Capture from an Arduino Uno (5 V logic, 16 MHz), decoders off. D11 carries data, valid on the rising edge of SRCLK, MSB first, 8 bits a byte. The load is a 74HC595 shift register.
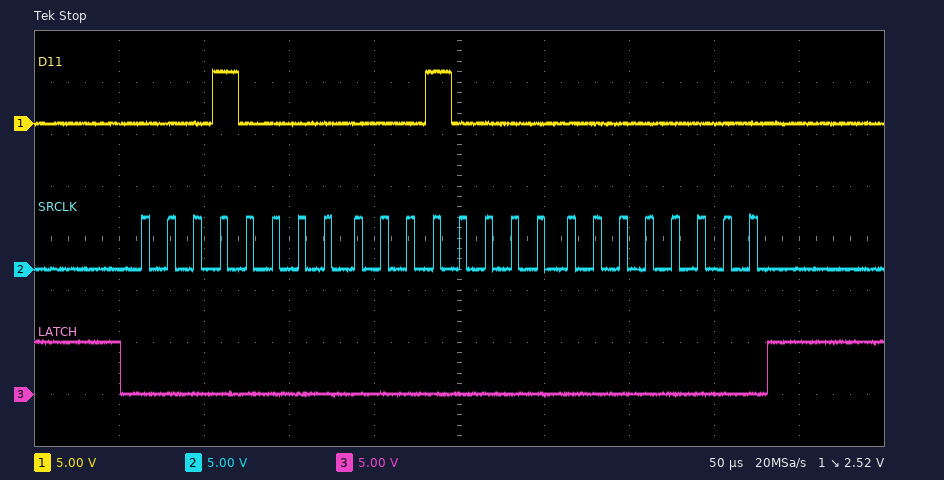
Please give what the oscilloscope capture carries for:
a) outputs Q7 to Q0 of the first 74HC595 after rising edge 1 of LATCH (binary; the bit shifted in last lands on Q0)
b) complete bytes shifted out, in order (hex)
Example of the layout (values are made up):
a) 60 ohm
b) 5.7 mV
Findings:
a) 00000000
b) 0x10 0x10 0x00
